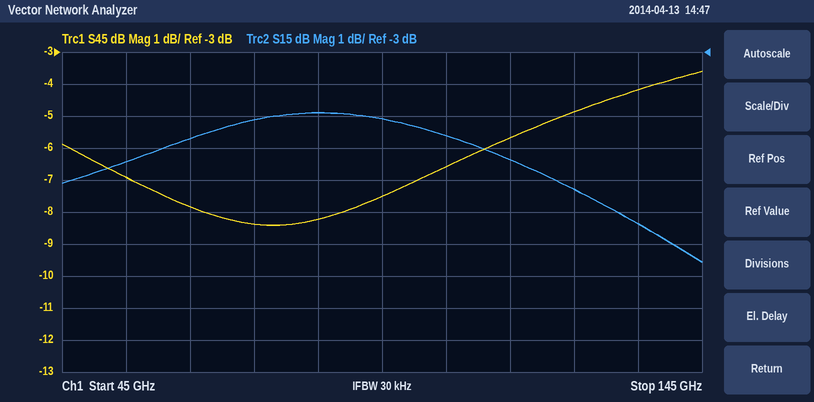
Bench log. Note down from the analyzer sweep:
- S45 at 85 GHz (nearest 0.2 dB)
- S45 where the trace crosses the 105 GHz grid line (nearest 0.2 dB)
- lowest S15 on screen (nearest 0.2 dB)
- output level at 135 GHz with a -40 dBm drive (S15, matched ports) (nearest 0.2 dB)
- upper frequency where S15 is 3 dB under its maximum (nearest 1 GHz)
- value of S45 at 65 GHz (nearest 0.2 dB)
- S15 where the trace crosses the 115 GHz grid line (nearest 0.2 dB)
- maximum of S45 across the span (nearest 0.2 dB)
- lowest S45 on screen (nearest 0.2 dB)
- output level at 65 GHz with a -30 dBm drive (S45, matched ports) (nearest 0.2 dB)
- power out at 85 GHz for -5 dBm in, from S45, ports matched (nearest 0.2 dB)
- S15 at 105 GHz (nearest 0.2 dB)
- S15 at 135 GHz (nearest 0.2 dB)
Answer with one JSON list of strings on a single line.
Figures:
["-8.2 dB", "-6.6 dB", "-9.6 dB", "-48.4 dBm", "131 GHz", "-7.8 dB", "-6.4 dB", "-3.6 dB", "-8.4 dB", "-37.8 dBm", "-13.2 dBm", "-5.6 dB", "-8.4 dB"]
